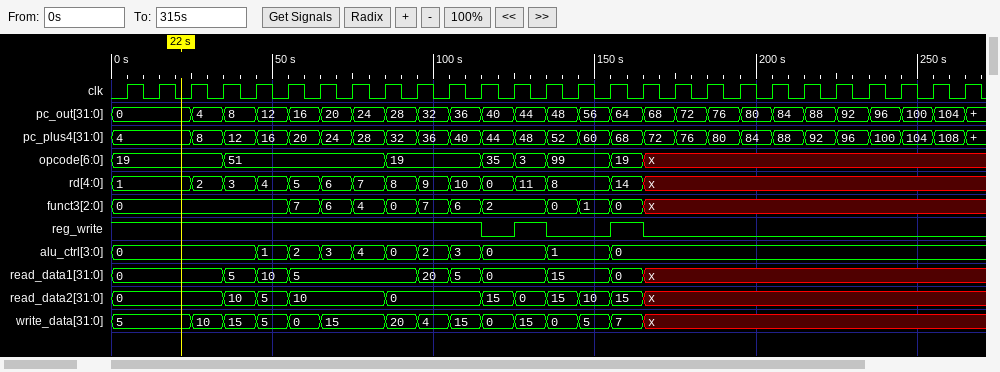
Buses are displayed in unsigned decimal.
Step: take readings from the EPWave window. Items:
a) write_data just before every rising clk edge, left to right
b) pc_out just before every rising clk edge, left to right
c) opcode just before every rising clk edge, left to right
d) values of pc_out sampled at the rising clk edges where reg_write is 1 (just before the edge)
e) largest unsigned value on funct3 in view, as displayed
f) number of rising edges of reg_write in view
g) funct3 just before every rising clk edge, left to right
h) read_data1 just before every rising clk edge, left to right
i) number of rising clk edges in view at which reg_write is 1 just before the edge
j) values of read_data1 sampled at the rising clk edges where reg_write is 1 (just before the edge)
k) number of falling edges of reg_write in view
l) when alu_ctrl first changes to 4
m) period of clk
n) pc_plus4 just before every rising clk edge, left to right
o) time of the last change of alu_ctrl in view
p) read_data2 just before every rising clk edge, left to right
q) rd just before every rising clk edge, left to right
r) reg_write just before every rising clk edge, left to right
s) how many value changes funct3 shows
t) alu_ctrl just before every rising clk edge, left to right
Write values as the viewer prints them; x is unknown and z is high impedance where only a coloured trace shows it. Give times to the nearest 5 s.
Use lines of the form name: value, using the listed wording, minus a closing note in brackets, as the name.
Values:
write_data just before every rising clk edge, left to right: 5, 5, 5, 10, 15, 5, 0, 15, 15, 20, 4, 15, 0, 15, 0, 5, 7, x, x, x, x, x, x, x, x, x, x
pc_out just before every rising clk edge, left to right: 0, 0, 0, 4, 8, 12, 16, 20, 24, 28, 32, 36, 40, 44, 48, 56, 64, 68, 72, 76, 80, 84, 88, 92, 96, 100, 104
opcode just before every rising clk edge, left to right: 19, 19, 19, 19, 51, 51, 51, 51, 51, 19, 19, 19, 35, 3, 99, 99, 19, x, x, x, x, x, x, x, x, x, x
values of pc_out sampled at the rising clk edges where reg_write is 1: 0, 0, 0, 4, 8, 12, 16, 20, 24, 28, 32, 36, 44, 64
largest unsigned value on funct3 in view, as displayed: 7
number of rising edges of reg_write in view: 2
funct3 just before every rising clk edge, left to right: 0, 0, 0, 0, 0, 0, 7, 6, 4, 0, 7, 6, 2, 2, 0, 1, 0, x, x, x, x, x, x, x, x, x, x
read_data1 just before every rising clk edge, left to right: 0, 0, 0, 0, 5, 10, 5, 5, 5, 5, 20, 5, 0, 0, 15, 15, 0, x, x, x, x, x, x, x, x, x, x
number of rising clk edges in view at which reg_write is 1 just before the edge: 14
values of read_data1 sampled at the rising clk edges where reg_write is 1: 0, 0, 0, 0, 5, 10, 5, 5, 5, 5, 20, 5, 0, 0
number of falling edges of reg_write in view: 3
when alu_ctrl first changes to 4: 75 s
period of clk: 10 s
pc_plus4 just before every rising clk edge, left to right: 4, 4, 4, 8, 12, 16, 20, 24, 28, 32, 36, 40, 44, 48, 52, 60, 68, 72, 76, 80, 84, 88, 92, 96, 100, 104, 108
time of the last change of alu_ctrl in view: 155 s
read_data2 just before every rising clk edge, left to right: 0, 0, 0, 0, 10, 5, 10, 10, 10, 0, 0, 0, 15, 0, 15, 10, 15, x, x, x, x, x, x, x, x, x, x
rd just before every rising clk edge, left to right: 1, 1, 1, 2, 3, 4, 5, 6, 7, 8, 9, 10, 0, 11, 8, 8, 14, x, x, x, x, x, x, x, x, x, x
reg_write just before every rising clk edge, left to right: 1 1 1 1 1 1 1 1 1 1 1 1 0 1 0 0 1 0 0 0 0 0 0 0 0 0 0
how many value changes funct3 shows: 11
alu_ctrl just before every rising clk edge, left to right: 0, 0, 0, 0, 0, 1, 2, 3, 4, 0, 2, 3, 0, 0, 1, 1, 0, 0, 0, 0, 0, 0, 0, 0, 0, 0, 0
